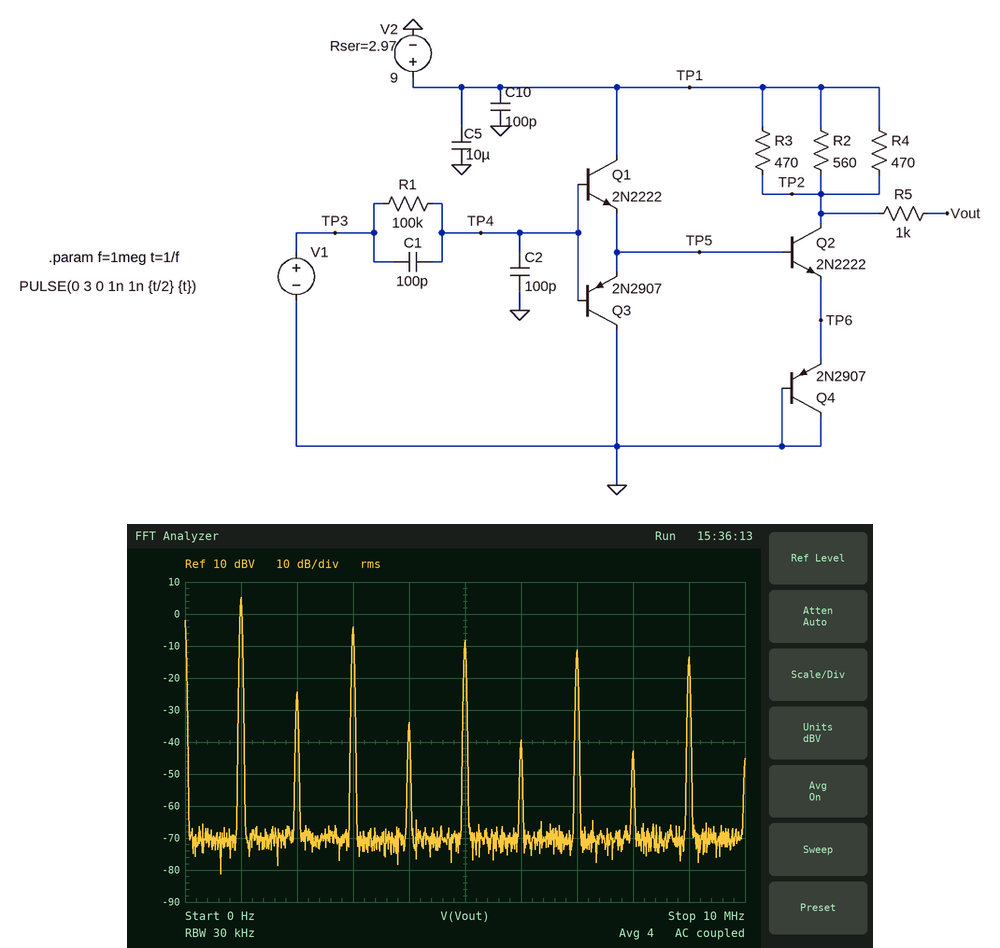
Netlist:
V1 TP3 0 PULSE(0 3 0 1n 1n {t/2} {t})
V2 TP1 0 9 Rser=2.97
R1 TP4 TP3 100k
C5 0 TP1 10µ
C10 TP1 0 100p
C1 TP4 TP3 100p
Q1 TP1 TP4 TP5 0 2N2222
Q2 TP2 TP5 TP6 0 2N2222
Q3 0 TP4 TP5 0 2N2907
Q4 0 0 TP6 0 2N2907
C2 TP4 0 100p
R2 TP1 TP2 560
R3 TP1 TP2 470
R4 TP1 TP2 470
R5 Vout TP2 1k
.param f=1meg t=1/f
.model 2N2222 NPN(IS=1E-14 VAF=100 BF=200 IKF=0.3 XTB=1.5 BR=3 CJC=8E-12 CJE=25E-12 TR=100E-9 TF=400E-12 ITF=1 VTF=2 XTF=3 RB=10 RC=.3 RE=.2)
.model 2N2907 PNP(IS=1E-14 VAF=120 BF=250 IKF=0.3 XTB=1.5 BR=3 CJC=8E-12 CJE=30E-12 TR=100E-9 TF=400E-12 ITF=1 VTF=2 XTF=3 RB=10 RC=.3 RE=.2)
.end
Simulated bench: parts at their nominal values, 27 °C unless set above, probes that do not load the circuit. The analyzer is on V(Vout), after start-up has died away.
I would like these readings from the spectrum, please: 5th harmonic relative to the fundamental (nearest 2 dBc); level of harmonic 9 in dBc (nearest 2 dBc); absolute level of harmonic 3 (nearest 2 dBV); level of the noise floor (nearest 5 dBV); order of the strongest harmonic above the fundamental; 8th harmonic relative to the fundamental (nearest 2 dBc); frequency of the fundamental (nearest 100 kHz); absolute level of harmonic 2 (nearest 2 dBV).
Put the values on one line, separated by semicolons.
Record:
-14 dBc; -18 dBc; -4 dBV; -70 dBV; 3; -48 dBc; 1.0 MHz; -24 dBV
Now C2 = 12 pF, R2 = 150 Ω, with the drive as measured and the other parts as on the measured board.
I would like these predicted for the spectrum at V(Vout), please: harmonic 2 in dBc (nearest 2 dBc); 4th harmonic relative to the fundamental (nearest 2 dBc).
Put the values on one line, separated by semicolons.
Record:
-48 dBc; -46 dBc
